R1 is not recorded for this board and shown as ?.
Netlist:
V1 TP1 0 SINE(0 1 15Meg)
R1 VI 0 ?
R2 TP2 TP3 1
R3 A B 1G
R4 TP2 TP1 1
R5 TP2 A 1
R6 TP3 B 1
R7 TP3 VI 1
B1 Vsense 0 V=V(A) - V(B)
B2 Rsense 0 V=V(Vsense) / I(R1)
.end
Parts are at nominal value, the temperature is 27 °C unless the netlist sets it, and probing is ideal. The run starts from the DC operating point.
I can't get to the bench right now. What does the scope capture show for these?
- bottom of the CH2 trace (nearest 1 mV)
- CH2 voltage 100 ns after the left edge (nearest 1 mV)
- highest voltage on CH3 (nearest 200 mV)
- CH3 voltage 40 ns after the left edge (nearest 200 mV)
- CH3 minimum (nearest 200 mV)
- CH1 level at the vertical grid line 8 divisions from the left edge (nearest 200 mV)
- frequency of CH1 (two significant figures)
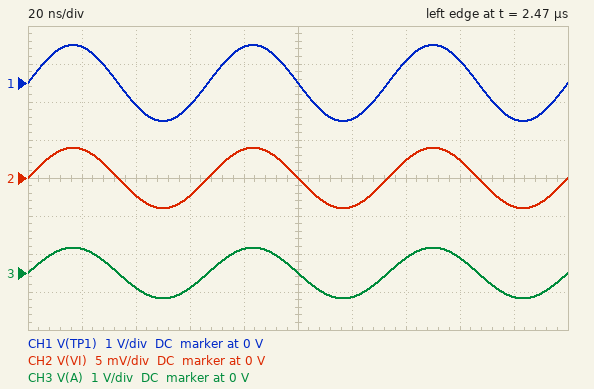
-4 mV
0 V
600 mV
-400 mV
-600 mV
600 mV
15 MHz
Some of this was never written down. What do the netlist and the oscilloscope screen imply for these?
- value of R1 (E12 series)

0.012 Ω
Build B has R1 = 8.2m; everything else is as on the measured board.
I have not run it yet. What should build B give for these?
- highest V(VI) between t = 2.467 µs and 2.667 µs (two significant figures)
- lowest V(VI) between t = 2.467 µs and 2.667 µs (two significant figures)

2.7 mV
-2.7 mV
